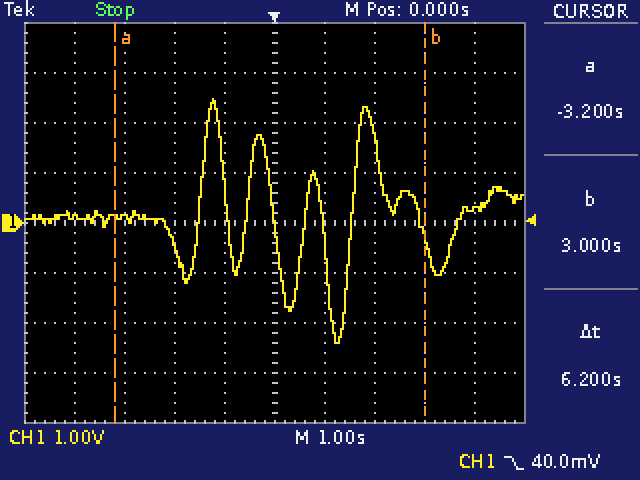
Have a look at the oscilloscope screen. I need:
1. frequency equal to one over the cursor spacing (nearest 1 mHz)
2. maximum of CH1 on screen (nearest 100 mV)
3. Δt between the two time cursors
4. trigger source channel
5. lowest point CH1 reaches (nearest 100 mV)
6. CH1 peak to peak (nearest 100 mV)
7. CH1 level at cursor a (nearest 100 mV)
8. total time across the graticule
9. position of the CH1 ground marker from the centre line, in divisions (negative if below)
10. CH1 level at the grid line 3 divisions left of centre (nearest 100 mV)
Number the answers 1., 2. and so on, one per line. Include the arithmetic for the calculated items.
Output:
1. 1 / 6.2 s ≈ 161 mHz
2. 2.5 V
3. 6.2 s
4. CH1
5. -2.4 V
6. 2.5 V − (-2.4 V) = 4.9 V
7. 100 mV
8. 10 s
9. 0.0 div
10. 100 mV
